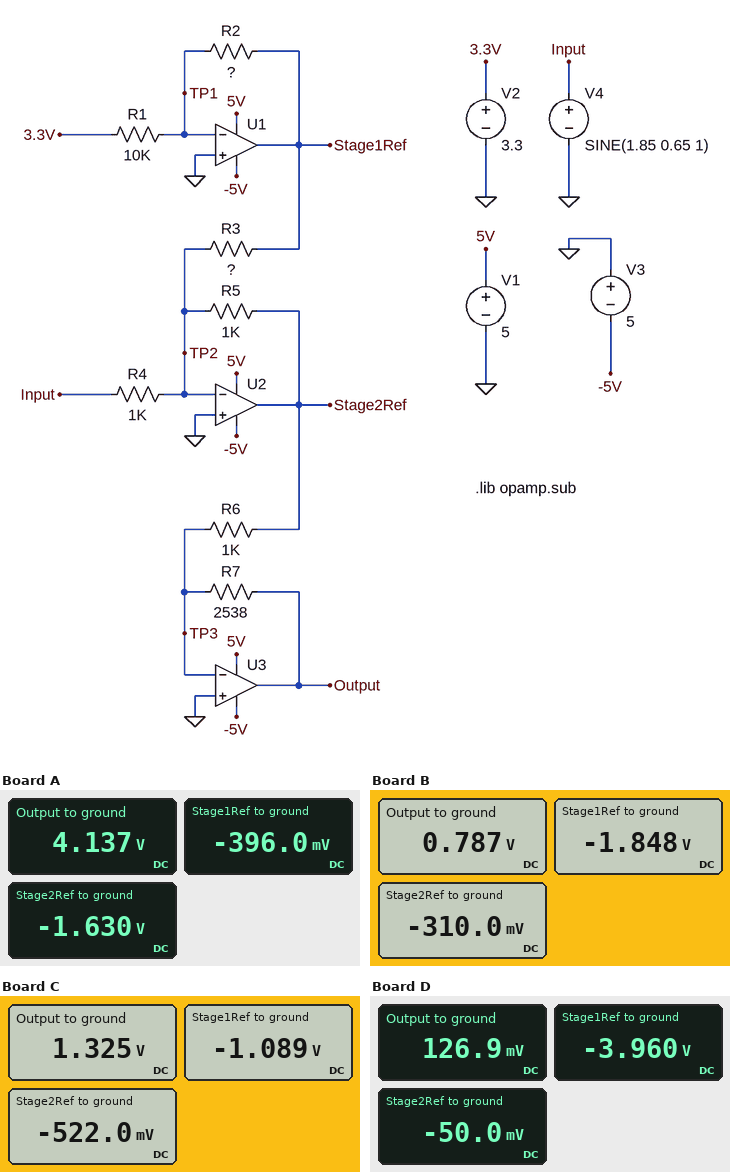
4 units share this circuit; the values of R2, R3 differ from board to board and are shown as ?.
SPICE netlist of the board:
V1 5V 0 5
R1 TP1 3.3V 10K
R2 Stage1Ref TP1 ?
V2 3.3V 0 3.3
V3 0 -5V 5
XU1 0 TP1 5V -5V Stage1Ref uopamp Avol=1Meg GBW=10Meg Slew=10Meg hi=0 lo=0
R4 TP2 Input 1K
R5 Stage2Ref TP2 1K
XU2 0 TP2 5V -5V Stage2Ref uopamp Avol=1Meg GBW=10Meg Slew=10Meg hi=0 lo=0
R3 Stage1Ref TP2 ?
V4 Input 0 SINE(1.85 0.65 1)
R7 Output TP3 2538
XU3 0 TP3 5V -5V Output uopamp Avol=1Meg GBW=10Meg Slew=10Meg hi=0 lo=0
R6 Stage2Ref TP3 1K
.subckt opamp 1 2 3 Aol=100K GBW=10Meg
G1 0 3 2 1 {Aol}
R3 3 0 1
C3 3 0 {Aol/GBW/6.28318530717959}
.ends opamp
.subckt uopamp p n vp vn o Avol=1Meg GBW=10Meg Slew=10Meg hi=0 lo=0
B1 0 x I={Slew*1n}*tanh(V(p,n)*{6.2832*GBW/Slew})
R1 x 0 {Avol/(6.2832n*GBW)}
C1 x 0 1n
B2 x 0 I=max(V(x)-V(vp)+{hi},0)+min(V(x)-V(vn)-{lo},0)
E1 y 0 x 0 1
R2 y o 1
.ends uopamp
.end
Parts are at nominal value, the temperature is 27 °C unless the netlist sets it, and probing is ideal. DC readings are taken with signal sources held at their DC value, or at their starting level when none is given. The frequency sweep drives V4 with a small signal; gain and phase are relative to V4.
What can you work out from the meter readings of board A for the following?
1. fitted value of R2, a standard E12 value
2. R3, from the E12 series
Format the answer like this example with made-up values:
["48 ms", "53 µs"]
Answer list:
["1.2 kΩ", "1.8 kΩ"]
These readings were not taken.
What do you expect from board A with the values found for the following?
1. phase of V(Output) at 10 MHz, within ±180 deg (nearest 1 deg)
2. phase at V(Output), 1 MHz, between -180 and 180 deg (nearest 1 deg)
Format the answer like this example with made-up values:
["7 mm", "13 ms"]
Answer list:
["-143 deg", "-34 deg"]
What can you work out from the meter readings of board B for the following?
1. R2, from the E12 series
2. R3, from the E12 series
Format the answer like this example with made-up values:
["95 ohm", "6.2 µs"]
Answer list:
["5.6 kΩ", "1.2 kΩ"]
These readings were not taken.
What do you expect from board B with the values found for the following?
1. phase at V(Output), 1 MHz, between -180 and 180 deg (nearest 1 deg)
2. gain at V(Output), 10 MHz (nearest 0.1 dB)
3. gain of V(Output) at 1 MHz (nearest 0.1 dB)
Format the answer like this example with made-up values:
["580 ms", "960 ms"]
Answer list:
["-35 deg", "-12.8 dB", "7.2 dB"]
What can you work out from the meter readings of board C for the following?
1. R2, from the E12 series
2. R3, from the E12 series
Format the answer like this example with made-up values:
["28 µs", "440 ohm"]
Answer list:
["3.3 kΩ", "820 Ω"]
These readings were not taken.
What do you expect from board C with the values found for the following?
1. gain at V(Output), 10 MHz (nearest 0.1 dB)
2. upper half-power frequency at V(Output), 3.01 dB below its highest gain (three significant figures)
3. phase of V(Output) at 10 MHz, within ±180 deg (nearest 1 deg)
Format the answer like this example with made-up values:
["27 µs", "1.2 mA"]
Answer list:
["-13.8 dB", "1.90 MHz", "-147 deg"]
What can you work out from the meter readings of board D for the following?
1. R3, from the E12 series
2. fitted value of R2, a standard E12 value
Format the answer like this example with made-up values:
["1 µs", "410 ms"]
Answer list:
["2.2 kΩ", "12 kΩ"]
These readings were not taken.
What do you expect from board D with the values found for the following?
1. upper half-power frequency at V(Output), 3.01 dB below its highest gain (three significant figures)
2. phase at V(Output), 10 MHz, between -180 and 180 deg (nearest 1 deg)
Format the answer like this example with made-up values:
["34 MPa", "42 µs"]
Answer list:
["2.13 MHz", "-142 deg"]
